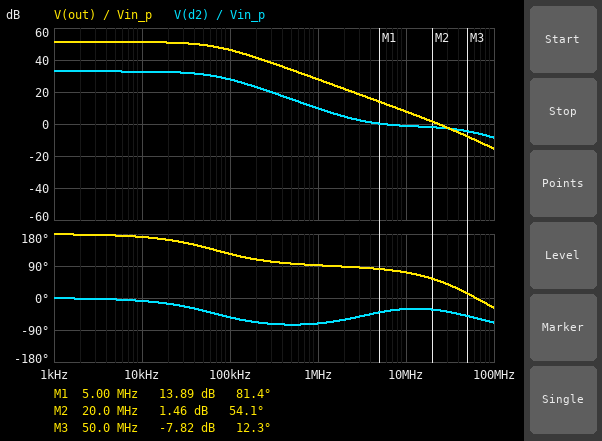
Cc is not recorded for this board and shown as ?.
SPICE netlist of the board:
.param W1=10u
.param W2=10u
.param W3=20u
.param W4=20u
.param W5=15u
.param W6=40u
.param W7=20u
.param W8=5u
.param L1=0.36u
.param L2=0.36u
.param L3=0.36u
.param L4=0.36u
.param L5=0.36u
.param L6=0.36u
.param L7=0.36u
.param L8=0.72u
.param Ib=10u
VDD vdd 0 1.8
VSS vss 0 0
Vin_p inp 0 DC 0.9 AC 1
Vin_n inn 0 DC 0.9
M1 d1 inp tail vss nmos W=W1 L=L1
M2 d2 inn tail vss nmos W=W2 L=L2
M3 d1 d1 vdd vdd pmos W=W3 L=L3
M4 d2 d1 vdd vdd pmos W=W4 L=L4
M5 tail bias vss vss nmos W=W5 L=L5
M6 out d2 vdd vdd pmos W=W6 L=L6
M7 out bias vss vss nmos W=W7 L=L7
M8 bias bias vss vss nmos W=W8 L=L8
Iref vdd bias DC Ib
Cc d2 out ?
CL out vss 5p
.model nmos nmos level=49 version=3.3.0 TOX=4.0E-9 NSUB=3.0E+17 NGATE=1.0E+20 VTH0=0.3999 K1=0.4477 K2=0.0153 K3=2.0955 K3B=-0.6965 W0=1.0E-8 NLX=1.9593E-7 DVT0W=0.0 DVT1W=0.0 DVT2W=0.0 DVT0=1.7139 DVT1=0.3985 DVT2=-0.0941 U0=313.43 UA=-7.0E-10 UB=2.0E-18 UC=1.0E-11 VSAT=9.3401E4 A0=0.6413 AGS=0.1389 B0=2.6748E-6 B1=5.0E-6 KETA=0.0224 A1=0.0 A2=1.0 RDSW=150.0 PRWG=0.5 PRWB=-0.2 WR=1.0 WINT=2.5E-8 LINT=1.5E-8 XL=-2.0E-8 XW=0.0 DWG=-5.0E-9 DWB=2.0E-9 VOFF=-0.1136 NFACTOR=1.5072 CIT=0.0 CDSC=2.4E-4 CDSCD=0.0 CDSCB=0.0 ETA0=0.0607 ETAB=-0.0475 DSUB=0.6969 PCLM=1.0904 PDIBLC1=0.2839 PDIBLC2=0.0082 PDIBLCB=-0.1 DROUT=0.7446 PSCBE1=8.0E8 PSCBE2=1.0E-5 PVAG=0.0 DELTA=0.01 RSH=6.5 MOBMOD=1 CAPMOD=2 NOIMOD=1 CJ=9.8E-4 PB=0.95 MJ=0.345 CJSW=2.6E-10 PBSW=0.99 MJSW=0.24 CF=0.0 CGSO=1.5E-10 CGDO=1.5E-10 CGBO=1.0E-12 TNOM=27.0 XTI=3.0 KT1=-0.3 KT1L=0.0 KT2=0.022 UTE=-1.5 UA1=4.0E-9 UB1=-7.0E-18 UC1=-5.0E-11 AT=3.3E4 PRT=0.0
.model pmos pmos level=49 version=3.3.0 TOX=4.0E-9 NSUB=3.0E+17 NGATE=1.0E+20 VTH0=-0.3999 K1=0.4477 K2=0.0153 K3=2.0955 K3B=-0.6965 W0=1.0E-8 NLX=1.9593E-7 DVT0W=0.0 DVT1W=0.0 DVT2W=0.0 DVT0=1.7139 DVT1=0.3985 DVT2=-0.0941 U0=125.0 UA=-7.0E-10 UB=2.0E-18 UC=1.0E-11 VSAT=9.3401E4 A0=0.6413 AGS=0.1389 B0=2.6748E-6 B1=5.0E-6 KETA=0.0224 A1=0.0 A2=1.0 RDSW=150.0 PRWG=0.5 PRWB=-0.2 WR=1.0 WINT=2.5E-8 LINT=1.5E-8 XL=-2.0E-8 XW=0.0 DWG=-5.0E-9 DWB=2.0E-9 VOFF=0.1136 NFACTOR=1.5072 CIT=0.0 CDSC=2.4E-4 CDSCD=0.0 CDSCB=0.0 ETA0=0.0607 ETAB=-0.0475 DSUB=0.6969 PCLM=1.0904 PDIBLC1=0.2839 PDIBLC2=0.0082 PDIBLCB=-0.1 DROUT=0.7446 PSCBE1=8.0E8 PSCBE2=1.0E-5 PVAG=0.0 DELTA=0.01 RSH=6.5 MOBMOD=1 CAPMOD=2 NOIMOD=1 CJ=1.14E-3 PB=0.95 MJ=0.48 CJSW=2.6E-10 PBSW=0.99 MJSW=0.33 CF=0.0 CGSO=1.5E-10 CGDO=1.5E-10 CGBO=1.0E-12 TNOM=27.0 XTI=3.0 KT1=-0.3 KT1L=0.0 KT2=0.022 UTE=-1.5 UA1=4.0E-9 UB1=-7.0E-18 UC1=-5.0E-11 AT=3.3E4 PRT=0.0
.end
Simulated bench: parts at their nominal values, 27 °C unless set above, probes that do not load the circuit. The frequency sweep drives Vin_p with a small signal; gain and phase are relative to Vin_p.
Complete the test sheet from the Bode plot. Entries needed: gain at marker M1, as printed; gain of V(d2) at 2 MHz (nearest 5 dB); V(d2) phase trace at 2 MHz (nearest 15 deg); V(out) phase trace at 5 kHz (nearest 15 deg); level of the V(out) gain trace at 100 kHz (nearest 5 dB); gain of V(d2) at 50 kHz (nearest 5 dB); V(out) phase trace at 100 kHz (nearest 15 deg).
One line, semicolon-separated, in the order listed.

13.89 dB; 5 dB; -60 deg; 180 deg; 45 dB; 30 dB; 120 deg
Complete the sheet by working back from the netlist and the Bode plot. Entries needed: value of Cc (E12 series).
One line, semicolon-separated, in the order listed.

2.7 pF
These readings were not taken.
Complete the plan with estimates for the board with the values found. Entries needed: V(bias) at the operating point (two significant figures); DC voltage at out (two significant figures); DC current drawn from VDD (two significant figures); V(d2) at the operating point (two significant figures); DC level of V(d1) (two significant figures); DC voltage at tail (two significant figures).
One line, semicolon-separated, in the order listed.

540 mV; 110 mV; 130 µA; 1.0 V; 1.0 V; 320 mV
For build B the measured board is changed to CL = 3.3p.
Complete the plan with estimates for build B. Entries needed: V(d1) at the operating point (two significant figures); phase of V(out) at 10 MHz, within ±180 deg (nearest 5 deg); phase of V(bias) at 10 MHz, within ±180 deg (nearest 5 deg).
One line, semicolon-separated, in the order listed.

1.0 V; 75 deg; 160 deg
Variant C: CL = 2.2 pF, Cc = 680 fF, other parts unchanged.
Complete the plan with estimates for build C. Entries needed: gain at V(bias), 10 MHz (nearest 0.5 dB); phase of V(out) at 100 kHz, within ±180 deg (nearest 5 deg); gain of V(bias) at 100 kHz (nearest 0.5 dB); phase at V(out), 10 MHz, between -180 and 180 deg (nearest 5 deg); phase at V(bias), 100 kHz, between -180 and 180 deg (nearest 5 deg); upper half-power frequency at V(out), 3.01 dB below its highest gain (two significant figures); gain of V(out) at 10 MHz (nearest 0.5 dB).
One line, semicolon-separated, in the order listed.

-36.5 dB; 160 deg; -45.5 dB; 85 deg; -110 deg; 260 kHz; 19.5 dB
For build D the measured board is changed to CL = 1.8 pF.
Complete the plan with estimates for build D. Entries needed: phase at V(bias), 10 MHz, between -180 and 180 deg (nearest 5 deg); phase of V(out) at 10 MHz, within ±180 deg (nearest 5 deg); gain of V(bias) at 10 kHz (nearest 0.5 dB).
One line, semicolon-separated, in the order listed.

160 deg; 80 deg; -65.0 dB
